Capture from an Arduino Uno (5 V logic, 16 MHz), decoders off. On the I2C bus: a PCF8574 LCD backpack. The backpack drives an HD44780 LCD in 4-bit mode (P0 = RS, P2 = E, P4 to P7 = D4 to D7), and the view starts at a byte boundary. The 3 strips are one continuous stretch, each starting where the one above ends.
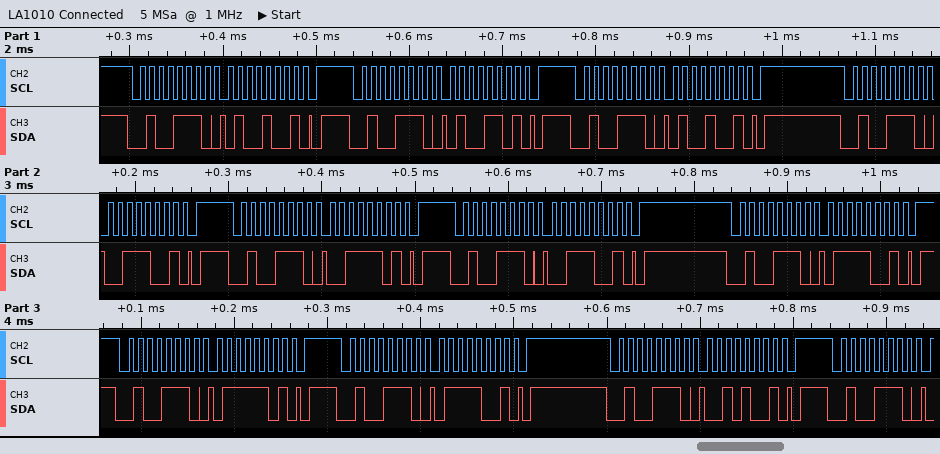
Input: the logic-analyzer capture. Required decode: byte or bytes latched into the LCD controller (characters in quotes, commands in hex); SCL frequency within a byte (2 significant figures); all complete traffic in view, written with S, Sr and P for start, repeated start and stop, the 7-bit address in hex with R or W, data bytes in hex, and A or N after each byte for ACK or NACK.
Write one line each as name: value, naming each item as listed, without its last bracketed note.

byte or bytes latched into the LCD controller: 'C'
SCL frequency within a byte: 100 kHz
all complete traffic in view, written with S, Sr and P for start, repeated start and stop, the 7-bit address in hex with R or W, data bytes in hex, and A or N after each byte for ACK or NACK: S 27W A 49 A P S 27W A 4D A P S 27W A 49 A P S 27W A 39 A P S 27W A 3D A P S 27W A 39 A P S 27W A 79 A P S 27W A 7D A P S 27W A 79 A P S 27W A 29 A P S 27W A
